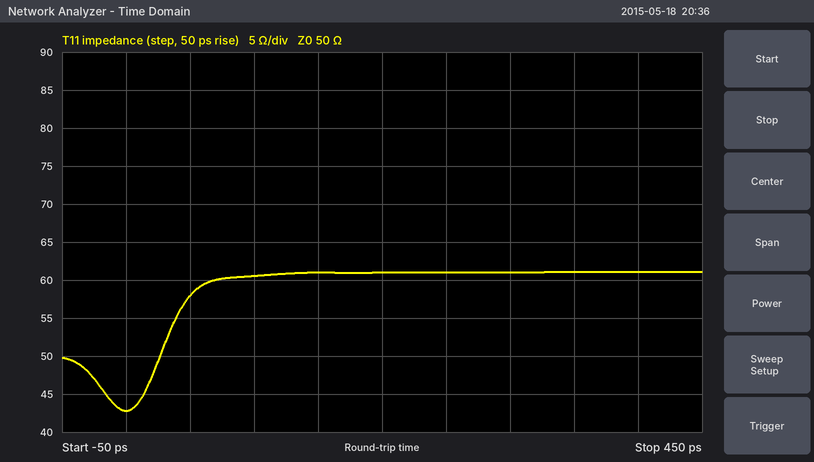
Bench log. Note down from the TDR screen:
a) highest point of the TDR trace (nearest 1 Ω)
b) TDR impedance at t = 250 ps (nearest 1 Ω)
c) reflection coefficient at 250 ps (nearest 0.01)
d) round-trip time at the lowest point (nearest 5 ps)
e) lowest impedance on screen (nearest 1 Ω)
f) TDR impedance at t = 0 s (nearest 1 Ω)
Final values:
61 Ω
61 Ω
+0.10
0 ps
43 Ω
43 Ω
